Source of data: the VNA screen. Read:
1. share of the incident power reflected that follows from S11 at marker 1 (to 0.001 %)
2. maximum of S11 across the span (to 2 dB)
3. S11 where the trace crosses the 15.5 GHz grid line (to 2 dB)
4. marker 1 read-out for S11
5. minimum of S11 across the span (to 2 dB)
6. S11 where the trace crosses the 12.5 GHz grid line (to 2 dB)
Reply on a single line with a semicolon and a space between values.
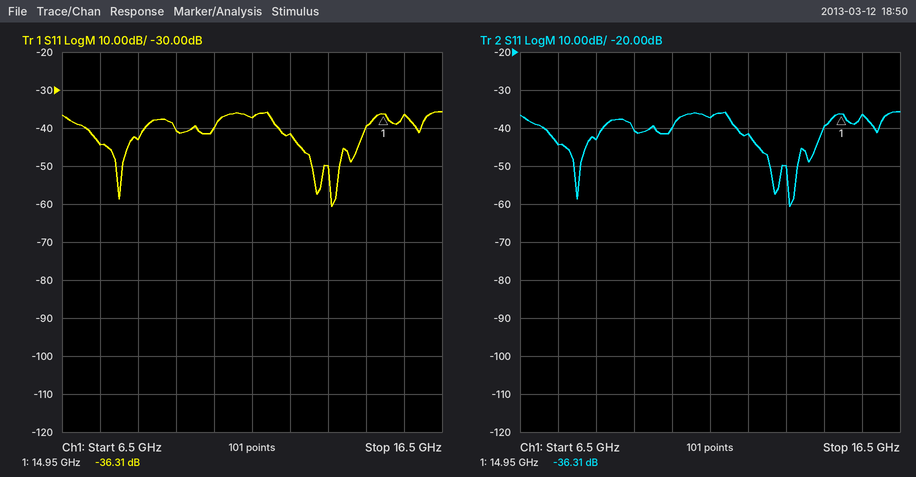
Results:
0.023 %; -36 dB; -36 dB; -36.31 dB; -60 dB; -42 dB
